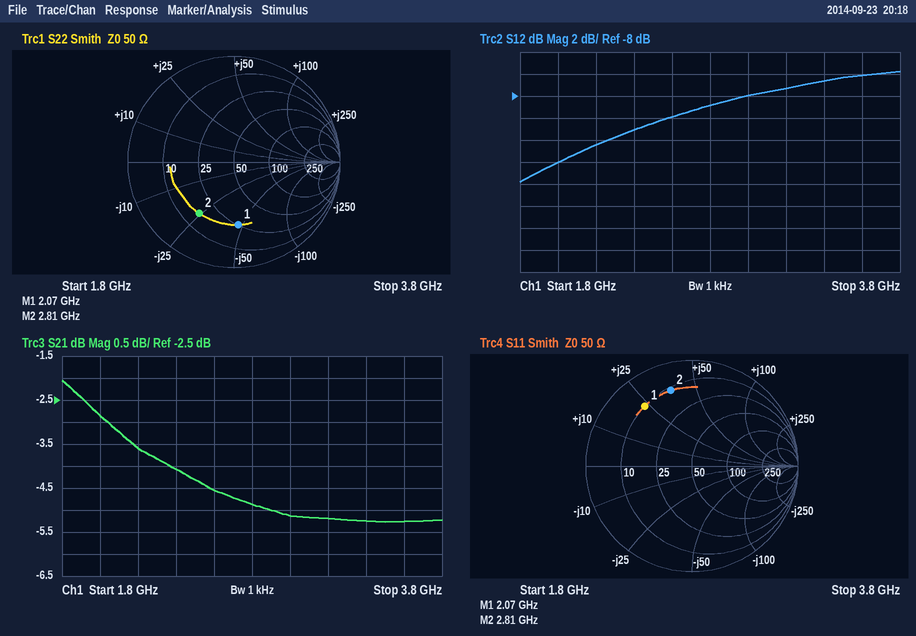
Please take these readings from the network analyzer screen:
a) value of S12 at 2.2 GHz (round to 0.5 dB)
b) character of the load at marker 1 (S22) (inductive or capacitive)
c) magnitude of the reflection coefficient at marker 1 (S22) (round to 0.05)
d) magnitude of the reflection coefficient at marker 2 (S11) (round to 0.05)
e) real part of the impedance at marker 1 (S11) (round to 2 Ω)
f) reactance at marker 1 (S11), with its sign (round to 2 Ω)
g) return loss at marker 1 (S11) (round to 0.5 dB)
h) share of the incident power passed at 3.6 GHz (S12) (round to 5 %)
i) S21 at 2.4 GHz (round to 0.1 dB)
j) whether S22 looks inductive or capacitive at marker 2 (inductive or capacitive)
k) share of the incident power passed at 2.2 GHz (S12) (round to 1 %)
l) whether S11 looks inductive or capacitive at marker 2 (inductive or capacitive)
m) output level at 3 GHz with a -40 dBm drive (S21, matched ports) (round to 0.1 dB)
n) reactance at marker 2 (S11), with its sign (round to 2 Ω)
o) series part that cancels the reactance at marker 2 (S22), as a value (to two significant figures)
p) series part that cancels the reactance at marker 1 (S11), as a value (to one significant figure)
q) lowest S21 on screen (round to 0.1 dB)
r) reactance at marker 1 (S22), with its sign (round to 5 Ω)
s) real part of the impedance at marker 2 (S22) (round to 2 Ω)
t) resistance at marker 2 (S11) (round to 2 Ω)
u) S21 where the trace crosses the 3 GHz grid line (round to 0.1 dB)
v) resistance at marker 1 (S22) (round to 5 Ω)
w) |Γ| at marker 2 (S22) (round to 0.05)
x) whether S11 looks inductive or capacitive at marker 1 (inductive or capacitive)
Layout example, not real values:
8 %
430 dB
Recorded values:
-12.5 dB
capacitive
0.60
0.75
10 Ω
+24 Ω
3.0 dB
25 %
-4.1 dB
capacitive
6 %
inductive
-45.1 dBm
+36 Ω
1.4 nH
3 pF
-5.3 dB
-45 Ω
16 Ω
12 Ω
-5.1 dB
25 Ω
0.60
inductive
